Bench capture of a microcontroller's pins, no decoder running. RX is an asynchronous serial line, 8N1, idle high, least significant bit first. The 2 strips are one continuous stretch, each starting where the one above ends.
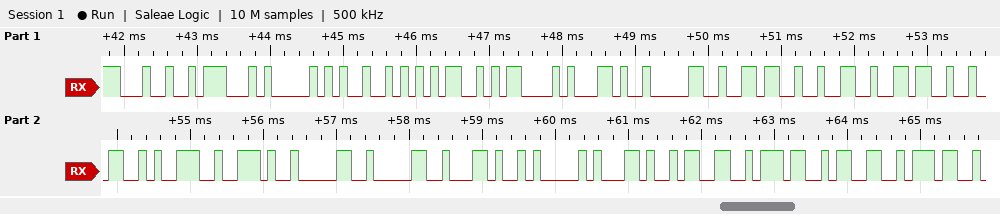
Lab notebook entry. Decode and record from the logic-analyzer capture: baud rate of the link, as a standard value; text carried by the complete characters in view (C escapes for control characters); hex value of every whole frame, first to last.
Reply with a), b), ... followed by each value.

a) 9600 baud
b) "$GPRMC,062629.00,A,3737"
c) 24 47 50 52 4D 43 2C 30 36 32 36 32 39 2E 30 30 2C 41 2C 33 37 33 37
